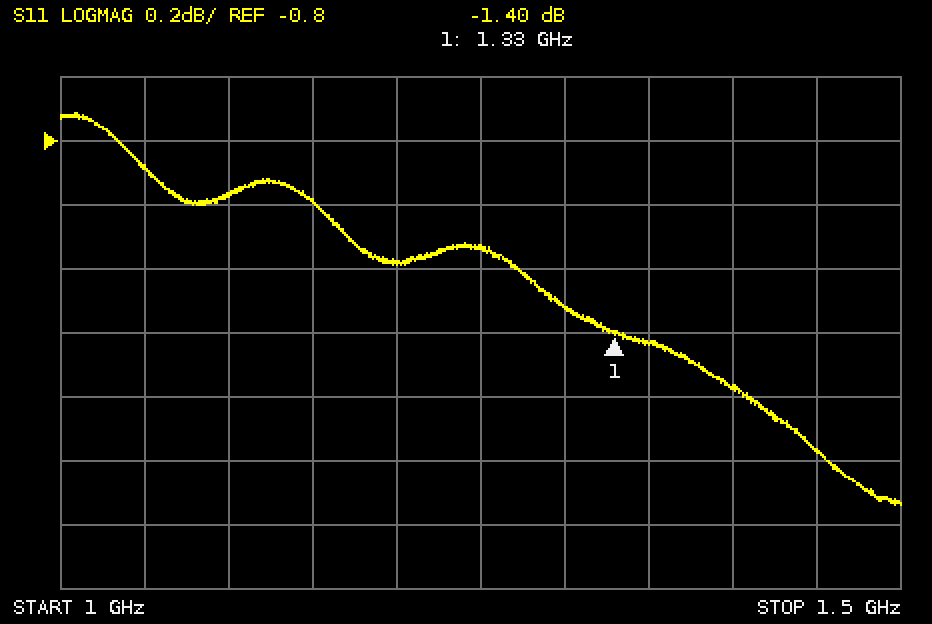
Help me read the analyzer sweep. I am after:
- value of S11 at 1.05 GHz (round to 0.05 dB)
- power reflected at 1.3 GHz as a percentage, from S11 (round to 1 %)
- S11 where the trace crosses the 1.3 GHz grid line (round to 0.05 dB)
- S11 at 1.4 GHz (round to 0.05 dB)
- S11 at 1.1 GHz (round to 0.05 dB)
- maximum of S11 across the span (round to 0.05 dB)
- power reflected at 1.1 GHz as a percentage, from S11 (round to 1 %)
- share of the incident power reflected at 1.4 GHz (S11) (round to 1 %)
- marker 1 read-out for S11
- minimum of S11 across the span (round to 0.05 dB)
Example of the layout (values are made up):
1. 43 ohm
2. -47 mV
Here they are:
1. -0.90 dB
2. 74 %
3. -1.30 dB
4. -1.55 dB
5. -0.95 dB
6. -0.70 dB
7. 80 %
8. 70 %
9. -1.40 dB
10. -1.95 dB
